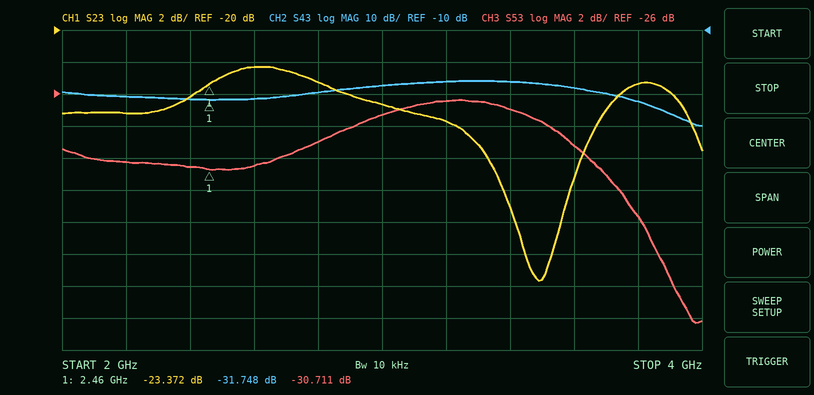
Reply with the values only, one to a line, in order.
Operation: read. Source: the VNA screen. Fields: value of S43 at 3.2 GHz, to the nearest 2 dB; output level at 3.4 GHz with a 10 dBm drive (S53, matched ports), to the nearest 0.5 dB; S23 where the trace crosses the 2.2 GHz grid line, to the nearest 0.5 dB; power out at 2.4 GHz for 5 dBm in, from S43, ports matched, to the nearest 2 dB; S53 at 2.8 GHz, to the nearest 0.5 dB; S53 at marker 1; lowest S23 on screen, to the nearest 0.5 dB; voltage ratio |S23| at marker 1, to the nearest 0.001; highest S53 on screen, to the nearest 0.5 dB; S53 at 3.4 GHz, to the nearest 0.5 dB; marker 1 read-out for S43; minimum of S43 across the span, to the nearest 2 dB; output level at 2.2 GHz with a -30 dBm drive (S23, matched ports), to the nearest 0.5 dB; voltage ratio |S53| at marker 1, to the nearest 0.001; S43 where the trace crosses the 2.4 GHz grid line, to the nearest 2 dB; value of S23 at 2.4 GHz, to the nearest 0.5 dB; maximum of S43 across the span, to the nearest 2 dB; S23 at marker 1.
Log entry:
-26 dB
-17.0 dBm
-25.0 dB
-26 dBm
-29.0 dB
-30.711 dB
-35.5 dB
0.068
-26.5 dB
-27.0 dB
-31.748 dB
-40 dB
-55.0 dBm
0.029
-32 dB
-24.0 dB
-26 dB
-23.372 dB
